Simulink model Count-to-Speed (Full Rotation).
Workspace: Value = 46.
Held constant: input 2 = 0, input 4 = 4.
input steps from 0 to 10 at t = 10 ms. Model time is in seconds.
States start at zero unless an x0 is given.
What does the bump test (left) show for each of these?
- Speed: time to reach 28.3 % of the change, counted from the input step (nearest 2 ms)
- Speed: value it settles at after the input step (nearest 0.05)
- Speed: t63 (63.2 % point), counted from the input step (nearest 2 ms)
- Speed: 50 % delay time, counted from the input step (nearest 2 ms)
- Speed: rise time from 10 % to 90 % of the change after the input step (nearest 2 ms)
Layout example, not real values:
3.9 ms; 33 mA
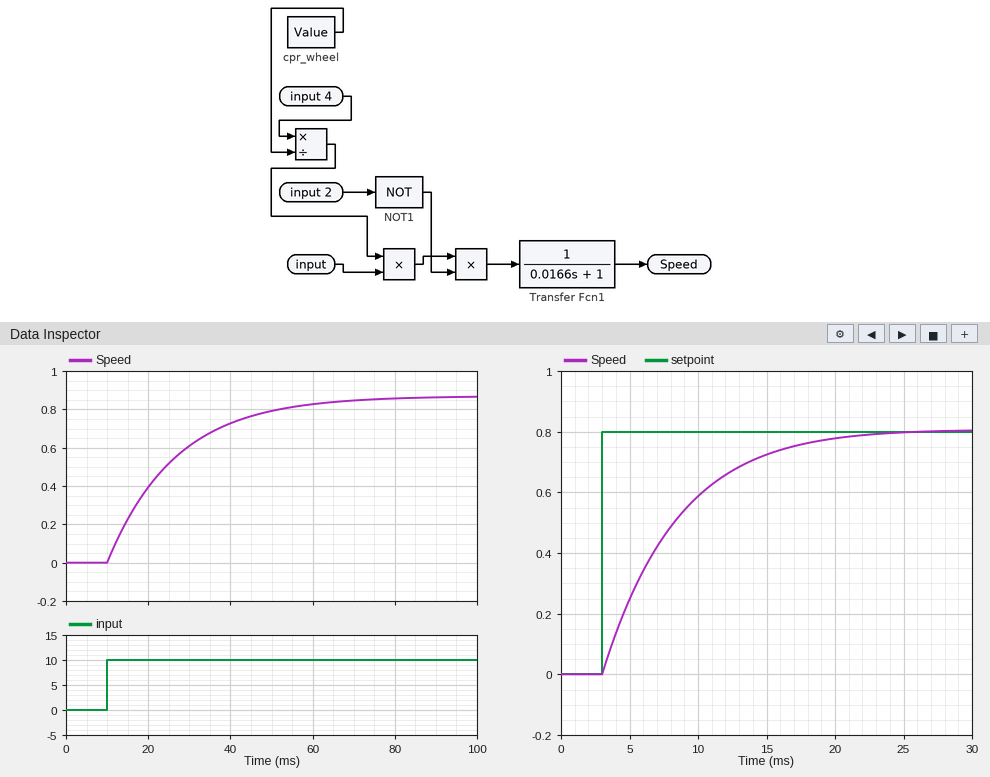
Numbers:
6 ms; 0.85; 16 ms; 12 ms; 36 ms
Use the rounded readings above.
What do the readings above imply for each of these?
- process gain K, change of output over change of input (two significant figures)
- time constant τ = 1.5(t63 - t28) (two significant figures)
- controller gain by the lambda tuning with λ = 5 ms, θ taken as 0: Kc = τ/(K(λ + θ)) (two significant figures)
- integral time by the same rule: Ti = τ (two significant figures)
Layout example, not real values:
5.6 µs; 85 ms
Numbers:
0.085; 15 ms; 35; 15 ms
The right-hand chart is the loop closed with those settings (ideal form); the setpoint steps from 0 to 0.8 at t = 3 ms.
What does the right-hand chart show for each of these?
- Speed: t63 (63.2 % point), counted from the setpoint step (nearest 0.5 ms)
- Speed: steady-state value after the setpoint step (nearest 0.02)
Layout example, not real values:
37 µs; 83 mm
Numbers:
5.5 ms; 0.80
